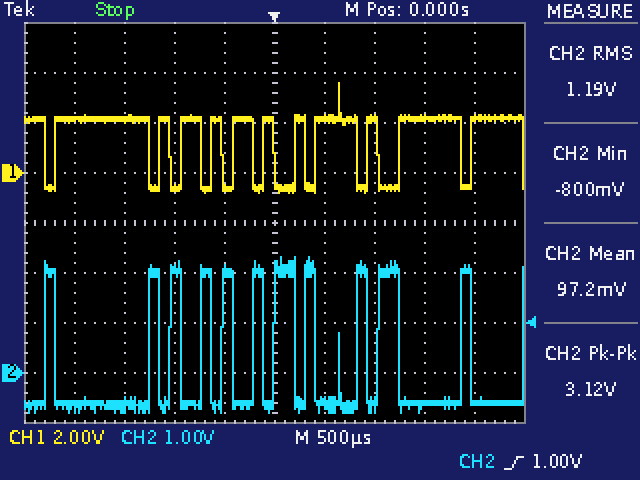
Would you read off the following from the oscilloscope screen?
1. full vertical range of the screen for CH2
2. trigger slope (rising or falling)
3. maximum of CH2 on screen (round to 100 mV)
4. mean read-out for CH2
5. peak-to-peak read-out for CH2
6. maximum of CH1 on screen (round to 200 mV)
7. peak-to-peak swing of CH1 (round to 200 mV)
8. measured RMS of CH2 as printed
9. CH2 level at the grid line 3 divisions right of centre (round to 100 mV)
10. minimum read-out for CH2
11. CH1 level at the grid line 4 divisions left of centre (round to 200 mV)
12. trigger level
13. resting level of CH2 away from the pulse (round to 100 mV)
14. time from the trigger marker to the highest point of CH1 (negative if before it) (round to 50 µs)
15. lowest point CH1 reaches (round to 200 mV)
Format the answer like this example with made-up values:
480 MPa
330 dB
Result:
8 V
rising
2.3 V
97.2 mV
3.12 V
3.6 V
4.4 V
1.19 V
-600 mV
-800 mV
2.2 V
1.00 V
-600 mV
+650 µs
-800 mV
